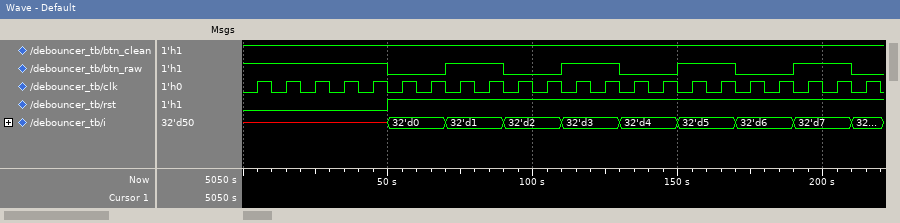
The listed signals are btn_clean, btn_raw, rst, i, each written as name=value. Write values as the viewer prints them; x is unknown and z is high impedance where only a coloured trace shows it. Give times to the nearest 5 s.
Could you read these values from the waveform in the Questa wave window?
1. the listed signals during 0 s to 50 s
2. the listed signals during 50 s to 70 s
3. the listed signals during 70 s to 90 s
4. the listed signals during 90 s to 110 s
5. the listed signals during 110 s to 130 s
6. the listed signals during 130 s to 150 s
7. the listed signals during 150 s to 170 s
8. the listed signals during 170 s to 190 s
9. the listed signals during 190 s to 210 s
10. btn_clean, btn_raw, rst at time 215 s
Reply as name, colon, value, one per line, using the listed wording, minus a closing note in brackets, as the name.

the listed signals during 0 s to 50 s: btn_clean=1, btn_raw=1, rst=0, i=x
the listed signals during 50 s to 70 s: btn_clean=1, btn_raw=0, rst=1, i=32'd0
the listed signals during 70 s to 90 s: btn_clean=1, btn_raw=1, rst=1, i=32'd1
the listed signals during 90 s to 110 s: btn_clean=1, btn_raw=0, rst=1, i=32'd2
the listed signals during 110 s to 130 s: btn_clean=1, btn_raw=1, rst=1, i=32'd3
the listed signals during 130 s to 150 s: btn_clean=1, btn_raw=0, rst=1, i=32'd4
the listed signals during 150 s to 170 s: btn_clean=1, btn_raw=1, rst=1, i=32'd5
the listed signals during 170 s to 190 s: btn_clean=1, btn_raw=0, rst=1, i=32'd6
the listed signals during 190 s to 210 s: btn_clean=1, btn_raw=1, rst=1, i=32'd7
btn_clean, btn_raw, rst at time 215 s: btn_clean=1, btn_raw=0, rst=1
